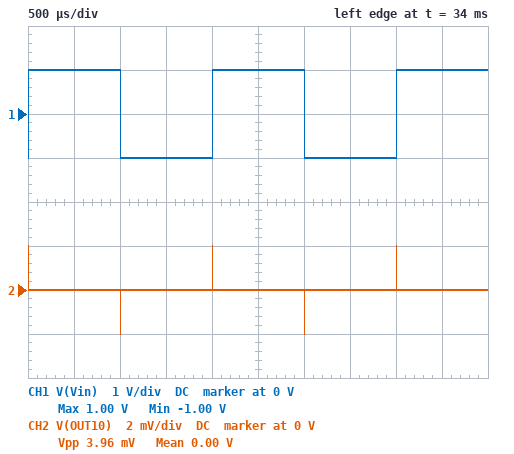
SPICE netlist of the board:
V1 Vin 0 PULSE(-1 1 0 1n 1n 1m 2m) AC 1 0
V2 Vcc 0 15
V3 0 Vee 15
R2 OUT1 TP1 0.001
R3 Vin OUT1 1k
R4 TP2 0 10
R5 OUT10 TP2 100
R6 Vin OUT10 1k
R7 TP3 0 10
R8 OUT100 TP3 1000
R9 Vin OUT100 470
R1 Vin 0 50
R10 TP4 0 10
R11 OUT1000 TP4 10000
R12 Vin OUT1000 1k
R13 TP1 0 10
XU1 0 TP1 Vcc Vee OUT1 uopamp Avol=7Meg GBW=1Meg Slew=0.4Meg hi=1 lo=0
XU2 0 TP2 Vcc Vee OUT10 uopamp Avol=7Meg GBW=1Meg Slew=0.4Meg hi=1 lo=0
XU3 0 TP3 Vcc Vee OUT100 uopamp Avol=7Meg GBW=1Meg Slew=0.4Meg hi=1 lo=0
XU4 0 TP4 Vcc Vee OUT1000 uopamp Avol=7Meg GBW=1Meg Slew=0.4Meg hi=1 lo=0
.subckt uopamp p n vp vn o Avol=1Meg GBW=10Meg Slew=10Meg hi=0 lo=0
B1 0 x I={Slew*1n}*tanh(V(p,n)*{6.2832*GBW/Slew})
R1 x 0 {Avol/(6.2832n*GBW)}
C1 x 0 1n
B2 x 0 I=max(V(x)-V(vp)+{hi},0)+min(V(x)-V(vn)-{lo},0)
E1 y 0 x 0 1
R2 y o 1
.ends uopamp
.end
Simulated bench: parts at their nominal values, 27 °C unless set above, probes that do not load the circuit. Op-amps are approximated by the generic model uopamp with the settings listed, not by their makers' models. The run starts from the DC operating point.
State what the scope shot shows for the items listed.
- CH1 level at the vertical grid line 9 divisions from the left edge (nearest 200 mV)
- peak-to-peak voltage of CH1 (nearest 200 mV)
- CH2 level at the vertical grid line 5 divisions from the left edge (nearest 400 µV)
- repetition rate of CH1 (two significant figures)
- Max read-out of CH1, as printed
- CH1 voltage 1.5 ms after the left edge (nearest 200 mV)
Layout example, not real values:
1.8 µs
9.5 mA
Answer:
1.0 V
2.0 V
0 V
500 Hz
1.00 V
-1.0 V
